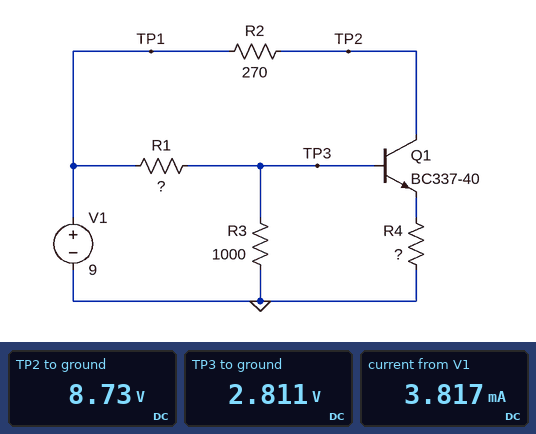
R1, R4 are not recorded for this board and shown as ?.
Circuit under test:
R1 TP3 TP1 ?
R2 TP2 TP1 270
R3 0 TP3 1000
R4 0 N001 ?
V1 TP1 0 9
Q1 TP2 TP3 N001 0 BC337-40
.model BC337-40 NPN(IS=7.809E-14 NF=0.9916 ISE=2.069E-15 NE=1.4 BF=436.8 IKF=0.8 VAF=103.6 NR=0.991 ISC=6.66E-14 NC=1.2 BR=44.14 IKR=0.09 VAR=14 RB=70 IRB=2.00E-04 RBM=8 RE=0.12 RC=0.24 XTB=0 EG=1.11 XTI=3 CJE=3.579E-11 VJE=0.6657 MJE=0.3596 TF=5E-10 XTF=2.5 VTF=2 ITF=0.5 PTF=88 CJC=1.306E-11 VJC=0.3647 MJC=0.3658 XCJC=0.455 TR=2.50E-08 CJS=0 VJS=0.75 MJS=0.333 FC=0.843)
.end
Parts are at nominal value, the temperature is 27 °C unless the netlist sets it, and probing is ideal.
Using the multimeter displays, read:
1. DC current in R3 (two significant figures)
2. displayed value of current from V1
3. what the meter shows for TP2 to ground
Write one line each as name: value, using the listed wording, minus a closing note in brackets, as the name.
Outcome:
DC current in R3: 2.8 mA
displayed value of current from V1: 3.817 mA
what the meter shows for TP2 to ground: 8.73 V
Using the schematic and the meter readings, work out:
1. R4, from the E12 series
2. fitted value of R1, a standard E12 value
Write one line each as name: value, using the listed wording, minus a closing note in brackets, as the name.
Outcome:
R4, from the E12 series: 2.2 kΩ
fitted value of R1, a standard E12 value: 2.2 kΩ
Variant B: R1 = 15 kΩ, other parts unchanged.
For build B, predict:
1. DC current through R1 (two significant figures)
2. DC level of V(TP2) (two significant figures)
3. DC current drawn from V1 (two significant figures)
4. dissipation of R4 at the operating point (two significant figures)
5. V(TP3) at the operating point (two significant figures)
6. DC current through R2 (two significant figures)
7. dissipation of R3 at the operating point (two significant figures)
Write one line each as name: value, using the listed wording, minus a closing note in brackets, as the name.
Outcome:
DC current through R1: 560 µA
DC level of V(TP2): 9.0 V
DC current drawn from V1: 590 µA
dissipation of R4 at the operating point: 1.6 µW
V(TP3) at the operating point: 560 mV
DC current through R2: 27 µA
dissipation of R3 at the operating point: 320 µW
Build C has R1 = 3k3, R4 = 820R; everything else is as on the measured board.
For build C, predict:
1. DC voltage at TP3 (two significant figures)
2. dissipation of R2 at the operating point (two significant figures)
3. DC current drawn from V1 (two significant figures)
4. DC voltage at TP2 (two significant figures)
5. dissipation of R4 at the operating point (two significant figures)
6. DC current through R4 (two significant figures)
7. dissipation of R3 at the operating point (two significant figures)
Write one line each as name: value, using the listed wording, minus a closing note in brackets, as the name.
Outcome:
DC voltage at TP3: 2.1 V
dissipation of R2 at the operating point: 870 µW
DC current drawn from V1: 3.9 mA
DC voltage at TP2: 8.5 V
dissipation of R4 at the operating point: 2.7 mW
DC current through R4: 1.8 mA
dissipation of R3 at the operating point: 4.4 mW
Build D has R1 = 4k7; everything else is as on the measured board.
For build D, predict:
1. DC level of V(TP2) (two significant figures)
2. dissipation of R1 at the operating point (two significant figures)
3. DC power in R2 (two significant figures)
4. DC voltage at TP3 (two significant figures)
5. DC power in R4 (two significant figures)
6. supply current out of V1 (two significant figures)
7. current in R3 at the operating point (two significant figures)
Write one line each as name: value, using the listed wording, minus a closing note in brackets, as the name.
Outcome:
DC level of V(TP2): 8.9 V
dissipation of R1 at the operating point: 12 mW
DC power in R2: 56 µW
DC voltage at TP3: 1.6 V
DC power in R4: 460 µW
supply current out of V1: 2.0 mA
current in R3 at the operating point: 1.6 mA
